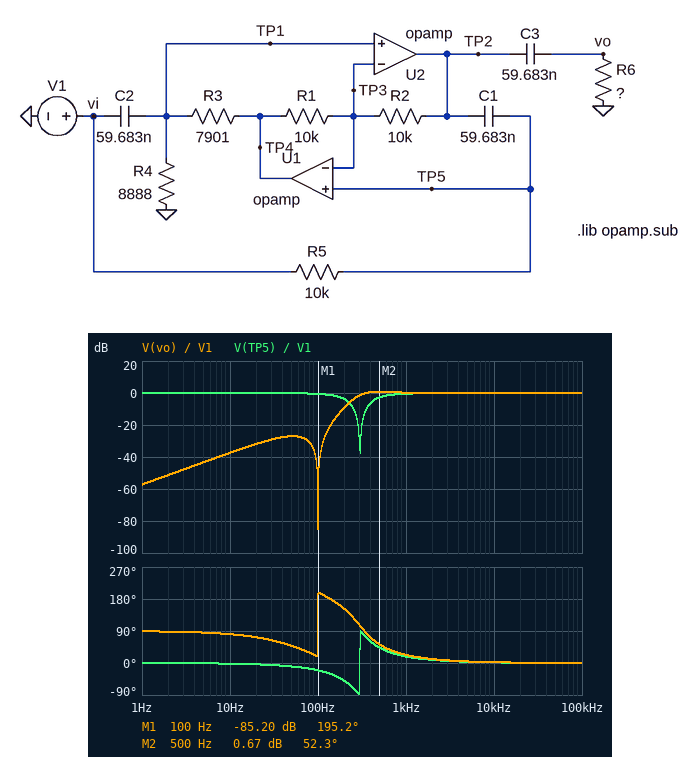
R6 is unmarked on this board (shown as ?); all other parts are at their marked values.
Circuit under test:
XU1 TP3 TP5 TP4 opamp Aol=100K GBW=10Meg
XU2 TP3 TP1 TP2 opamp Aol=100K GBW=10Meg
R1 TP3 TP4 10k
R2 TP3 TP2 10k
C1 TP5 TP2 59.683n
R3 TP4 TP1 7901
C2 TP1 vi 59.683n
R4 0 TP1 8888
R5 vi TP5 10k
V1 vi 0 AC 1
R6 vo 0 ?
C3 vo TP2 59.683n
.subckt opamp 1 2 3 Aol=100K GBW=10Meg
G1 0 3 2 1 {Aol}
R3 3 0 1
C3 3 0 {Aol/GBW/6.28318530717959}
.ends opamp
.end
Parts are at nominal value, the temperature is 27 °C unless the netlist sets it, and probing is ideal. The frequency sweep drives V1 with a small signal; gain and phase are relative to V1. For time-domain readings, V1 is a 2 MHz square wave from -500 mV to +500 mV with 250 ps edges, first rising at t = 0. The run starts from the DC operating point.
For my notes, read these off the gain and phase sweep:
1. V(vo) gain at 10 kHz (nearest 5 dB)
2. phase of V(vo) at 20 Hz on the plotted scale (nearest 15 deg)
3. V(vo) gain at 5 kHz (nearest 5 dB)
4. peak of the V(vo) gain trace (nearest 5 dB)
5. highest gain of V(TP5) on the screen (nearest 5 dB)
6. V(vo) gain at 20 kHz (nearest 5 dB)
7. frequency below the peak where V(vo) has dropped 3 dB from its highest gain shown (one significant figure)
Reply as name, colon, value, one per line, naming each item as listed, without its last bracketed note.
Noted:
V(vo) gain at 10 kHz: 0 dB
phase of V(vo) at 20 Hz on the plotted scale: 75 deg
V(vo) gain at 5 kHz: 0 dB
peak of the V(vo) gain trace: 0 dB
highest gain of V(TP5) on the screen: 0 dB
V(vo) gain at 20 kHz: 0 dB
frequency below the peak where V(vo) has dropped 3 dB from its highest gain shown: 300 Hz
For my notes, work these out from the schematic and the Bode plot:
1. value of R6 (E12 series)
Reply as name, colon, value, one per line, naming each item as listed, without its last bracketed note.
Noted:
value of R6: 33 kΩ
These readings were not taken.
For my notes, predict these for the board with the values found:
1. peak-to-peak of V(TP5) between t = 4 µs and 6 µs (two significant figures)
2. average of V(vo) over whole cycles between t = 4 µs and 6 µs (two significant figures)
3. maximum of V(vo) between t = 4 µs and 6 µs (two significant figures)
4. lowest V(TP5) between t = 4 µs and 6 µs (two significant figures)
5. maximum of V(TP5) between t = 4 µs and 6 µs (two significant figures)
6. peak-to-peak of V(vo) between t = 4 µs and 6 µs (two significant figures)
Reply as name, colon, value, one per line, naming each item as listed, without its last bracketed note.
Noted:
peak-to-peak of V(TP5) between t = 4 µs and 6 µs: 1.4 V
average of V(vo) over whole cycles between t = 4 µs and 6 µs: 490 mV
maximum of V(vo) between t = 4 µs and 6 µs: 1.2 V
lowest V(TP5) between t = 4 µs and 6 µs: -710 mV
maximum of V(TP5) between t = 4 µs and 6 µs: 700 mV
peak-to-peak of V(vo) between t = 4 µs and 6 µs: 1.4 V
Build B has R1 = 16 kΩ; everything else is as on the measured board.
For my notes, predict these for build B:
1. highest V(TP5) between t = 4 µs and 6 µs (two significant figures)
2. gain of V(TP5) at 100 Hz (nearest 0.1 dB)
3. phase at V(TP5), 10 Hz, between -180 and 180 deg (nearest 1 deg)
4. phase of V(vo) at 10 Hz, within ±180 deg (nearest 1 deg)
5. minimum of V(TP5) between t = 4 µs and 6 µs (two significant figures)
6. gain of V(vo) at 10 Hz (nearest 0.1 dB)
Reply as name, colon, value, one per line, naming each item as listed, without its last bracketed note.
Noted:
highest V(TP5) between t = 4 µs and 6 µs: 670 mV
gain of V(TP5) at 100 Hz: -0.2 dB
phase at V(TP5), 10 Hz, between -180 and 180 deg: -1 deg
phase of V(vo) at 10 Hz, within ±180 deg: 82 deg
minimum of V(TP5) between t = 4 µs and 6 µs: -680 mV
gain of V(vo) at 10 Hz: -25.3 dB
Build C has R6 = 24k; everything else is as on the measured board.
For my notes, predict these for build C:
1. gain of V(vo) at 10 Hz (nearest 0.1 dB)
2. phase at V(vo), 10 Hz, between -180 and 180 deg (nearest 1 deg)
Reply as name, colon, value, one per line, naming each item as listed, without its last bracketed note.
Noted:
gain of V(vo) at 10 Hz: -40.1 dB
phase at V(vo), 10 Hz, between -180 and 180 deg: 83 deg
